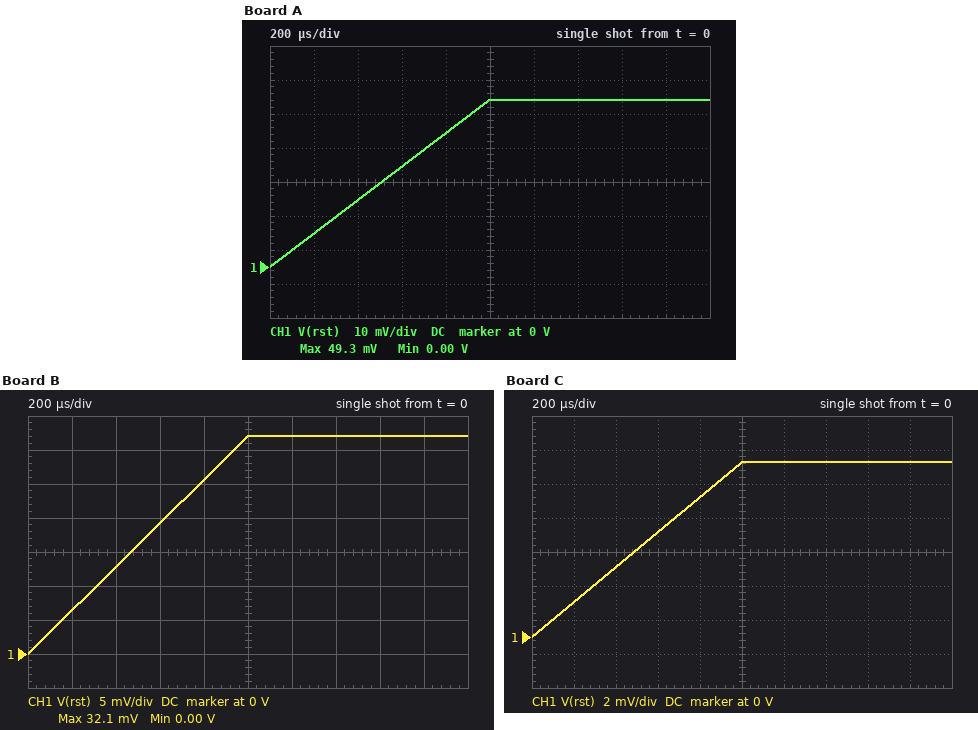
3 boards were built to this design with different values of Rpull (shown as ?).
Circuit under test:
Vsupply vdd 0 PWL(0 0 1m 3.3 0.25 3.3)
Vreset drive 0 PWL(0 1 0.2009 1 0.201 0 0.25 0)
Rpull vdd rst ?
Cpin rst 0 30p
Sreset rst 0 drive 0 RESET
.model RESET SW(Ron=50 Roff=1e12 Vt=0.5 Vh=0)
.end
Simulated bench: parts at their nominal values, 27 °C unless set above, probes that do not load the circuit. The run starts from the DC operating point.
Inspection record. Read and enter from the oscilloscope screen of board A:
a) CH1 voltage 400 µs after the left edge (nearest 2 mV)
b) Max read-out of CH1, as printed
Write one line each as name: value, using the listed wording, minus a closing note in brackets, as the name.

CH1 voltage 400 µs after the left edge: 20 mV
Max read-out of CH1, as printed: 49.3 mV
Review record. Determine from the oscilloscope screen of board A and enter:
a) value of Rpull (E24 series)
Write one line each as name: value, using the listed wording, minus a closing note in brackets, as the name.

value of Rpull: 3.3 kΩ
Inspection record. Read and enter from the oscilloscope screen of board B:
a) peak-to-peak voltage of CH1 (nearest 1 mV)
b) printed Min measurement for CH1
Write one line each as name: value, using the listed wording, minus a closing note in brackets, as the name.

peak-to-peak voltage of CH1: 32 mV
printed Min measurement for CH1: 0.00 V
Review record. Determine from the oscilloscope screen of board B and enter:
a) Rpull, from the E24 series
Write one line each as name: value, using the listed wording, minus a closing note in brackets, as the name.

Rpull, from the E24 series: 5.1 kΩ
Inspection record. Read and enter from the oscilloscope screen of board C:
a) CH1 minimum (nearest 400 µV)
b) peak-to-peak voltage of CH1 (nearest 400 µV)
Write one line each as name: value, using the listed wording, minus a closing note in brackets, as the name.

CH1 minimum: 0 V
peak-to-peak voltage of CH1: 10.4 mV
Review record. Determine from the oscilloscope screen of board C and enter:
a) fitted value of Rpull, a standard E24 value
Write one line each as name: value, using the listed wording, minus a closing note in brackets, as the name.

fitted value of Rpull, a standard E24 value: 16 kΩ
